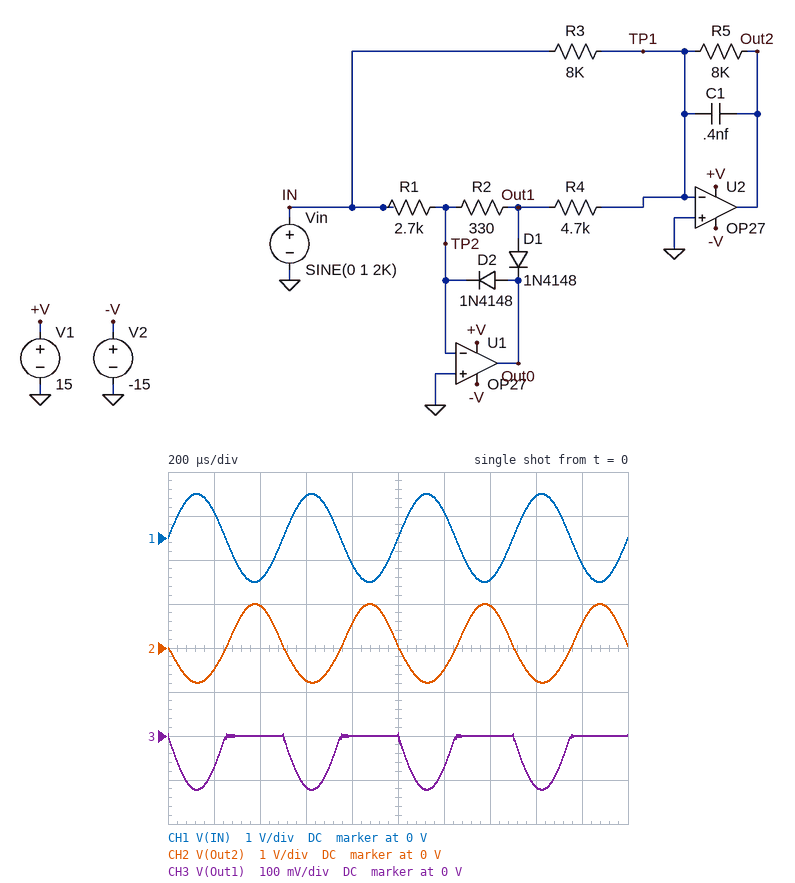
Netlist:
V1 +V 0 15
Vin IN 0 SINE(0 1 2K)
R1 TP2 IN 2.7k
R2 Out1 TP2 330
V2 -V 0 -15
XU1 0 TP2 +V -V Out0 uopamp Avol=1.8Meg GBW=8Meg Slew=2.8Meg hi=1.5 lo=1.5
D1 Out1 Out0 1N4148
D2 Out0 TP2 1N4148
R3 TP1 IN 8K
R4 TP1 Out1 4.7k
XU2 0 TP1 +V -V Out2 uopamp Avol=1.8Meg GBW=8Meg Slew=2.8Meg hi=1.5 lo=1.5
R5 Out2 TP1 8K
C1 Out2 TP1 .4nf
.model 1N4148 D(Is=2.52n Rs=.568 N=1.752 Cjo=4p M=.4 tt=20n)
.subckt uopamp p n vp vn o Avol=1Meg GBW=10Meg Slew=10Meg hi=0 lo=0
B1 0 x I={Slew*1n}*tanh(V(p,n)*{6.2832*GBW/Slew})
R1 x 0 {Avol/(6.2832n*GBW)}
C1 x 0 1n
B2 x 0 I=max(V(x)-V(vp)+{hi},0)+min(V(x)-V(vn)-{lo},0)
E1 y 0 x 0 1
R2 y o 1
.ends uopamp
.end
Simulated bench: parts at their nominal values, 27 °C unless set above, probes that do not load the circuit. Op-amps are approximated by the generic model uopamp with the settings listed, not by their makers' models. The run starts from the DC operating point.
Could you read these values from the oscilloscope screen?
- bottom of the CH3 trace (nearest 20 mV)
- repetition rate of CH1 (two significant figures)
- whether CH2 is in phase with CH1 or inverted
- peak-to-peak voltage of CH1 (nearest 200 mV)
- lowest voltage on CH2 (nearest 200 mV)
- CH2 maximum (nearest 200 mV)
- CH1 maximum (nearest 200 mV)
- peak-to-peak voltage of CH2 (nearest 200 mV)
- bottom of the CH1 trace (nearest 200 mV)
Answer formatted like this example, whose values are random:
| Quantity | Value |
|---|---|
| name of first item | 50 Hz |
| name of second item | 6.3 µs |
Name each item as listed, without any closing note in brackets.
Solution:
| Quantity | Value |
|---|---|
| bottom of the CH3 trace | -120 mV |
| repetition rate of CH1 | 2.0 kHz |
| whether CH2 is in phase with CH1 or inverted | inverted |
| peak-to-peak voltage of CH1 | 2.0 V |
| lowest voltage on CH2 | -800 mV |
| CH2 maximum | 1.0 V |
| CH1 maximum | 1.0 V |
| peak-to-peak voltage of CH2 | 1.8 V |
| bottom of the CH1 trace | -1.0 V |
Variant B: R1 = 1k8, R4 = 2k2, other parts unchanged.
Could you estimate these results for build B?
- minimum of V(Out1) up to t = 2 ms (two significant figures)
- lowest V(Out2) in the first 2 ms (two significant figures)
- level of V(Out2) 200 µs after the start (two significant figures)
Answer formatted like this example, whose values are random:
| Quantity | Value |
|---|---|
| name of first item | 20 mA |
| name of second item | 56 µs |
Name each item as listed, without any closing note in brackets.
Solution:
| Quantity | Value |
|---|---|
| minimum of V(Out1) up to t = 2 ms | -180 mV |
| lowest V(Out2) in the first 2 ms | -330 mV |
| level of V(Out2) 200 µs after the start | -210 mV |
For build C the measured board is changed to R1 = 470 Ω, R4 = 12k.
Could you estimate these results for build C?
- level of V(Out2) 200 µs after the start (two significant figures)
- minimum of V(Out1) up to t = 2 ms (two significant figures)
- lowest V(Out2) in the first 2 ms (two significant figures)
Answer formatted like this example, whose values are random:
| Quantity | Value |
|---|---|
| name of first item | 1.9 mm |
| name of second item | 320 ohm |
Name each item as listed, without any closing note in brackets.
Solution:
| Quantity | Value |
|---|---|
| level of V(Out2) 200 µs after the start | -330 mV |
| minimum of V(Out1) up to t = 2 ms | -700 mV |
| lowest V(Out2) in the first 2 ms | -530 mV |
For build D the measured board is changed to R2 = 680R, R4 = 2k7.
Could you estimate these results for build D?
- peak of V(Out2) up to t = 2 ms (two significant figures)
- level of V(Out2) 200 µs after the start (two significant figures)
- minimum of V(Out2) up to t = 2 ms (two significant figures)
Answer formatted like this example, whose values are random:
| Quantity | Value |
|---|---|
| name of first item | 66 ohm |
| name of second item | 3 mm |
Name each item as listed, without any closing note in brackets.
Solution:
| Quantity | Value |
|---|---|
| peak of V(Out2) up to t = 2 ms | 1.0 V |
| level of V(Out2) 200 µs after the start | -160 mV |
| minimum of V(Out2) up to t = 2 ms | -250 mV |
